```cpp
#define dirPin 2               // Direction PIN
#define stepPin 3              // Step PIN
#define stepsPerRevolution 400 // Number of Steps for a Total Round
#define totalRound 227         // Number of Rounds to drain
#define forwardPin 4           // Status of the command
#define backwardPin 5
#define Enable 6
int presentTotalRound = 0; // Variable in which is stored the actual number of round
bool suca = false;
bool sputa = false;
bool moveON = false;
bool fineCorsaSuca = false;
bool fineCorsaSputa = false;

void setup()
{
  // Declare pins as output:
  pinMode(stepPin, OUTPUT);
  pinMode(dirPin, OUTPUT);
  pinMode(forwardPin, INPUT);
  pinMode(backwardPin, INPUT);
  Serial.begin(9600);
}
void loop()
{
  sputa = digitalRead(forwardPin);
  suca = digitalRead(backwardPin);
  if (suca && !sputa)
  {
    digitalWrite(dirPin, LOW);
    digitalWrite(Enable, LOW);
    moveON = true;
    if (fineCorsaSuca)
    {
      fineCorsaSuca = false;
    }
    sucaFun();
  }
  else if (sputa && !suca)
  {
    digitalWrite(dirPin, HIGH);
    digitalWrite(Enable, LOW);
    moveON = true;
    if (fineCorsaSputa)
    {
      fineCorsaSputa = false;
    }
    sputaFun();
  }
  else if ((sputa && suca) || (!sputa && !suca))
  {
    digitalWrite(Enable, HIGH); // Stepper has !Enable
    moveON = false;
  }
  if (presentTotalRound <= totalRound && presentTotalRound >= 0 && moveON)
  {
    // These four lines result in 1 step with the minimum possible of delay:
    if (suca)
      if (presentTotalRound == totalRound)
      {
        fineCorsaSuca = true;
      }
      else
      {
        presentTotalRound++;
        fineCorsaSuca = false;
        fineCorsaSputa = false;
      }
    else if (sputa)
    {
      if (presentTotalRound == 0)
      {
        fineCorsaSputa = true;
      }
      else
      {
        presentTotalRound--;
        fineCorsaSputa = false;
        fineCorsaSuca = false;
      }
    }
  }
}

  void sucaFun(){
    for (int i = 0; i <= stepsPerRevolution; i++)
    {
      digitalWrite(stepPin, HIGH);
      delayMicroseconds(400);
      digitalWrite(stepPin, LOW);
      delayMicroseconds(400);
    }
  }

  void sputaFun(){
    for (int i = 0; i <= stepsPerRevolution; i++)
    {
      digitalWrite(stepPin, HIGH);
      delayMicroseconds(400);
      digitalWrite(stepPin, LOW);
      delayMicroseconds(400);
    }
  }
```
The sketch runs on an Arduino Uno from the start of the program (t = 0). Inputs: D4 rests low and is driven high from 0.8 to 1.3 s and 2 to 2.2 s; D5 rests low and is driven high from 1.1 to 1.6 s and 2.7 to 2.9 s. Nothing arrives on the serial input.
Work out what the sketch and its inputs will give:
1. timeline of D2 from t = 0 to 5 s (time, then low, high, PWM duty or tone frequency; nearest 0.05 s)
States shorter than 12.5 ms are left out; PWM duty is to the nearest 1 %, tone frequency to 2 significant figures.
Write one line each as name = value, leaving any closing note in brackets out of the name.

timeline of D2 from t = 0 to 5 s = 0 s low; 0.8 s high; 1.3 s low; 2 s high; 2.7 s low
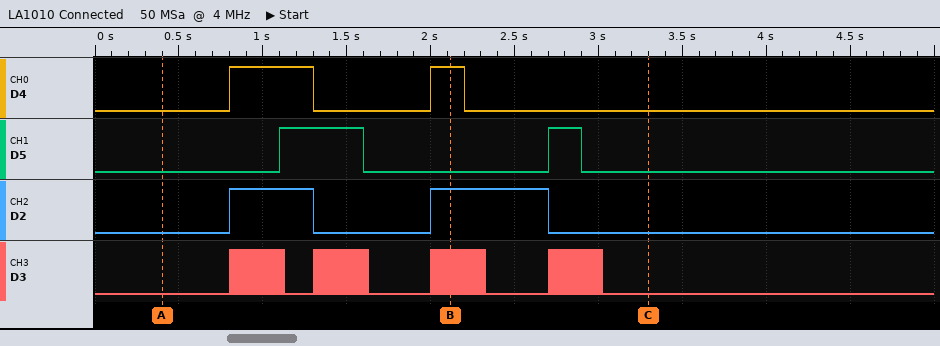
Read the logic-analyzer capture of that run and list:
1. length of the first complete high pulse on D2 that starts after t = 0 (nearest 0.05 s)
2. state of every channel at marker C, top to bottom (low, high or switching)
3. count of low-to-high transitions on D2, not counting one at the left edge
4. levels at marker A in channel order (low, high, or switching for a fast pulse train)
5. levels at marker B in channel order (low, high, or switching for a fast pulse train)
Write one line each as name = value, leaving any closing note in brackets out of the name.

length of the first complete high pulse on D2 that starts after t = 0 = 0.50 s
state of every channel at marker C, top to bottom = D4 low, D5 low, D2 low, D3 low
count of low-to-high transitions on D2, not counting one at the left edge = 2
levels at marker A in channel order = D4 low, D5 low, D2 low, D3 low
levels at marker B in channel order = D4 high, D5 low, D2 high, D3 switching
